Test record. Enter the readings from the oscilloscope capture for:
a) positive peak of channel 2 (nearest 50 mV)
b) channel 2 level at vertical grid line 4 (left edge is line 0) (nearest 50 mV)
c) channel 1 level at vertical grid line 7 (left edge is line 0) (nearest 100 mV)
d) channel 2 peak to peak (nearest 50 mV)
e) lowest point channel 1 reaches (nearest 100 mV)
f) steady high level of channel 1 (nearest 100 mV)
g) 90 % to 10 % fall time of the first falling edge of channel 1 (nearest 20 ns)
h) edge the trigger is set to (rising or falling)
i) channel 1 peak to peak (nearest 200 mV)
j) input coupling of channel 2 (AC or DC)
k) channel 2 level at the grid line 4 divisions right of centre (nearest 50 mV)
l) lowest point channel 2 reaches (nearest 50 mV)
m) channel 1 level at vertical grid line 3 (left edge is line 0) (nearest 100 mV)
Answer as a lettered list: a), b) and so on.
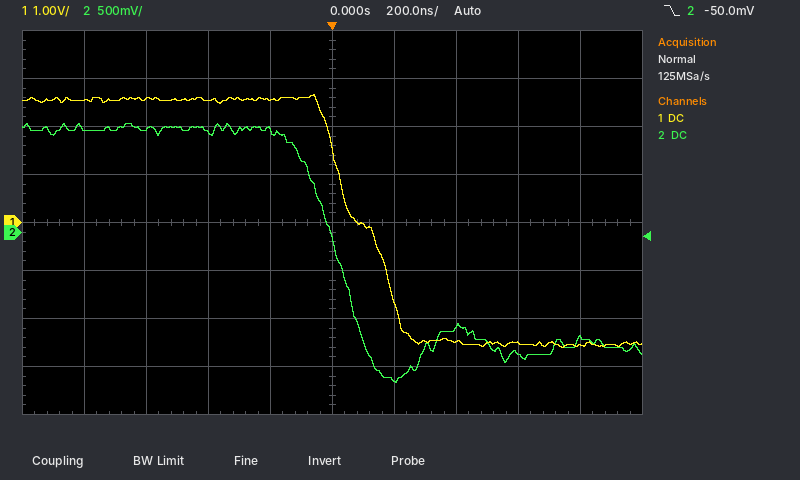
a) 1.15 V
b) 1.05 V
c) -2.5 V
d) 2.70 V
e) -2.6 V
f) 2.6 V
g) 240 ns
h) falling
i) 5.2 V
j) DC
k) -1.10 V
l) -1.55 V
m) 2.5 V
